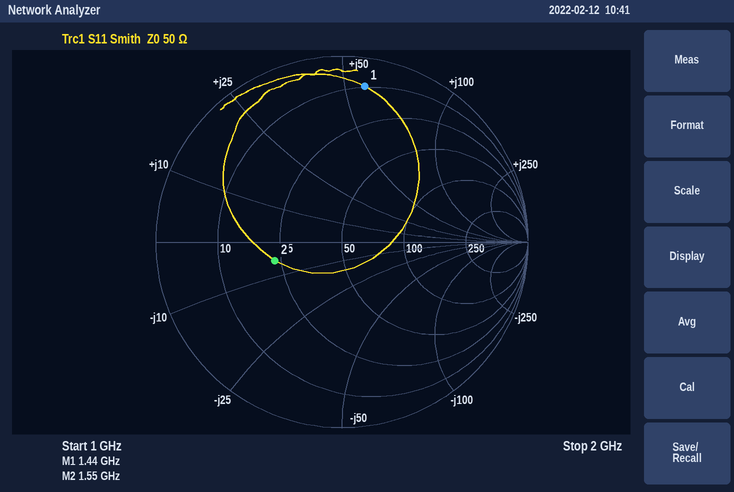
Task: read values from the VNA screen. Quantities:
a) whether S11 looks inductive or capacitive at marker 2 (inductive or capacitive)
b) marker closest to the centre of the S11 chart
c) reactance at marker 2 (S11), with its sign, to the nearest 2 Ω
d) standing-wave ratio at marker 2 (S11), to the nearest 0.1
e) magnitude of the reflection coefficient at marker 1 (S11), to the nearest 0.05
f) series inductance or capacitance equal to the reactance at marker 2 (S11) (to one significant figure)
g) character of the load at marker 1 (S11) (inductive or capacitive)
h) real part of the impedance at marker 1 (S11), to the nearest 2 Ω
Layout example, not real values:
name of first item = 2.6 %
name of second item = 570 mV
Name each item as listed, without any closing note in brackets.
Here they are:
whether S11 looks inductive or capacitive at marker 2 = capacitive
marker closest to the centre of the S11 chart = marker 2
reactance at marker 2 (S11), with its sign, to the nearest 2 Ω = -6 Ω
standing-wave ratio at marker 2 (S11), to the nearest 0.1 = 2.2
magnitude of the reflection coefficient at marker 1 (S11), to the nearest 0.05 = 0.85
series inductance or capacitance equal to the reactance at marker 2 (S11) = 20 pF
character of the load at marker 1 (S11) = inductive
real part of the impedance at marker 1 (S11), to the nearest 2 Ω = 10 Ω
